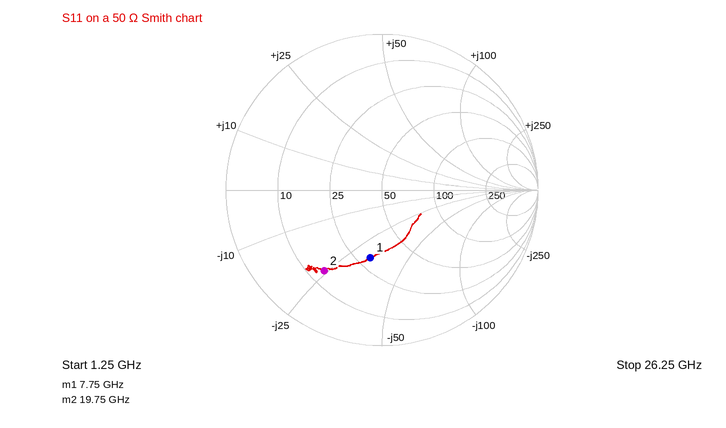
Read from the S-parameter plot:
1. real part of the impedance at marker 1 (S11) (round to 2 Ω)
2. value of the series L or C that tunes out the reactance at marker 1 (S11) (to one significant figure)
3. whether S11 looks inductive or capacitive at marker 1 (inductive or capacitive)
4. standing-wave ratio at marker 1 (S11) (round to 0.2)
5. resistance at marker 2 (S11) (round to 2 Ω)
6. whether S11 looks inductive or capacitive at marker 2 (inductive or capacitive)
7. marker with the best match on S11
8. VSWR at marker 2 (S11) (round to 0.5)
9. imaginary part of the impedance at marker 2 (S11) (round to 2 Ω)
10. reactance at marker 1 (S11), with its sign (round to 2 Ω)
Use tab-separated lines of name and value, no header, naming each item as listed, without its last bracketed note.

real part of the impedance at marker 1 (S11)	30 Ω
value of the series L or C that tunes out the reactance at marker 1 (S11)	700 pH
whether S11 looks inductive or capacitive at marker 1	capacitive
standing-wave ratio at marker 1 (S11)	2.6
resistance at marker 2 (S11)	14 Ω
whether S11 looks inductive or capacitive at marker 2	capacitive
marker with the best match on S11	marker 1
VSWR at marker 2 (S11)	4.5
imaginary part of the impedance at marker 2 (S11)	-24 Ω
reactance at marker 1 (S11), with its sign	-32 Ω
